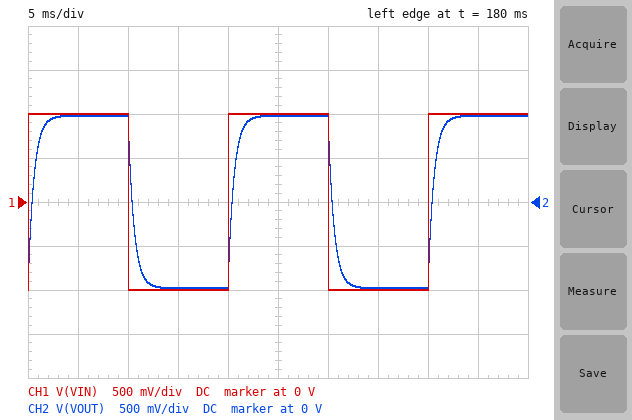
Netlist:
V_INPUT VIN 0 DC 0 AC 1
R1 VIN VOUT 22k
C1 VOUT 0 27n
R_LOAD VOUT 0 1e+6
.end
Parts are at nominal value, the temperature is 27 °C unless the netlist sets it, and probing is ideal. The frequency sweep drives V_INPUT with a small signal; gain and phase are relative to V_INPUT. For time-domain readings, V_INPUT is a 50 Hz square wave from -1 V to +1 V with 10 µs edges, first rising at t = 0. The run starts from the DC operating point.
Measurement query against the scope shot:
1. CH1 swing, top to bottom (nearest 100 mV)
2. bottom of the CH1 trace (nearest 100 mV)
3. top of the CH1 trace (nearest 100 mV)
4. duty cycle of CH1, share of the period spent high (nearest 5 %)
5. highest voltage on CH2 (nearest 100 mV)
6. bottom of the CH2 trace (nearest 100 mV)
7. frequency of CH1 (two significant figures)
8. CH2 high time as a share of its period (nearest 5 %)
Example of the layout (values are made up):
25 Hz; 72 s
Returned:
2.0 V; -1.0 V; 1.0 V; 50 %; 1.0 V; -1.0 V; 50 Hz; 50 %
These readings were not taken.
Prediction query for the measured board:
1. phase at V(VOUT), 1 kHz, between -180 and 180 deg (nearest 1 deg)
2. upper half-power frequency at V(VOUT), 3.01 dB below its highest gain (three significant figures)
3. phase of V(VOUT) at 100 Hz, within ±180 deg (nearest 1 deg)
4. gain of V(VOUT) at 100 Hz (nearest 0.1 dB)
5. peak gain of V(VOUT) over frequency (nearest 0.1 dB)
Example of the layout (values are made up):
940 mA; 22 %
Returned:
-75 deg; 274 Hz; -20 deg; -0.7 dB; -0.2 dB
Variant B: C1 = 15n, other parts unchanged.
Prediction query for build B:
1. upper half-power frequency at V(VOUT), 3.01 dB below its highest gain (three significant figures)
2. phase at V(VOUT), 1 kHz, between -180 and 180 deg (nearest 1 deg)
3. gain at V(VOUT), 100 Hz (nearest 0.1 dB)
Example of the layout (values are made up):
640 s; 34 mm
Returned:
493 Hz; -64 deg; -0.4 dB
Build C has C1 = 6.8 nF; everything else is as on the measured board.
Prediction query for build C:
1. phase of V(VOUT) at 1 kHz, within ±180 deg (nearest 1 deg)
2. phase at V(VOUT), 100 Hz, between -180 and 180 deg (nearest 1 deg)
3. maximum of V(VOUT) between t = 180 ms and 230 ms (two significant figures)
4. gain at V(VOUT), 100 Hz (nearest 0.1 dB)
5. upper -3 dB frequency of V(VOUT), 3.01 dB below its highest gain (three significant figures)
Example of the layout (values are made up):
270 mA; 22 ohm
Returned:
-43 deg; -5 deg; 980 mV; -0.2 dB; 1.09 kHz
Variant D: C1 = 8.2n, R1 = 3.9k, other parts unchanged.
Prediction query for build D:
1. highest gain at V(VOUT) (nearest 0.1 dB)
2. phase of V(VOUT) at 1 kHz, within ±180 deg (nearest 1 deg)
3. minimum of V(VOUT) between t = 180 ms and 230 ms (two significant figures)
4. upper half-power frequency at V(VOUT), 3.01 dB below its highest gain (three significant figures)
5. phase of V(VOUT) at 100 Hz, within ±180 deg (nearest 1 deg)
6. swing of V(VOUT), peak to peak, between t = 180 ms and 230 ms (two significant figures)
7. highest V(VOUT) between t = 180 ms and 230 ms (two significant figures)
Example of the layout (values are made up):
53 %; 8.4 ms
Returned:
0 dB; -11 deg; -1.0 V; 5.00 kHz; -1 deg; 2.0 V; 1.0 V
